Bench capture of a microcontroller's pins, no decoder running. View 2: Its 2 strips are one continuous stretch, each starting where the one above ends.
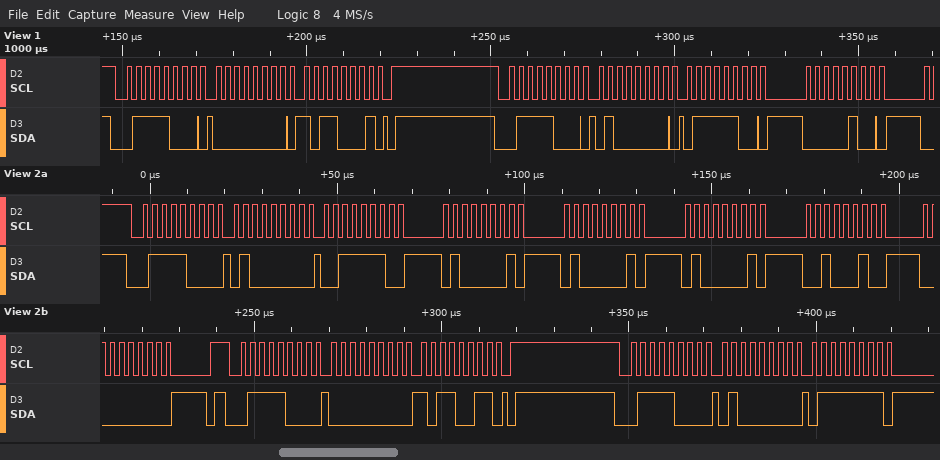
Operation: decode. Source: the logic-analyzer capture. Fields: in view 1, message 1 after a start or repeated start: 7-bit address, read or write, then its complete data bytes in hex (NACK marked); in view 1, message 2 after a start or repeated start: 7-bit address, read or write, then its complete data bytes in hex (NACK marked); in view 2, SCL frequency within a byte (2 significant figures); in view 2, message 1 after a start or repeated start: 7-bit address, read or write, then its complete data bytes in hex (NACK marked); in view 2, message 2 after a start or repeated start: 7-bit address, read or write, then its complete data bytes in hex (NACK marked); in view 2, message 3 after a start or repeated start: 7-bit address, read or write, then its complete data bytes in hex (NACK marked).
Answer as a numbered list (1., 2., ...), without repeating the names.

1. 0x3C write: 00 B1
2. 0x3C write: 40 7C 04
3. 400 kHz
4. 0x3C write: 40 3E 41 41 41 22 00
5. 0x3C write: 00 B3
6. 0x3C write: 40 7F
